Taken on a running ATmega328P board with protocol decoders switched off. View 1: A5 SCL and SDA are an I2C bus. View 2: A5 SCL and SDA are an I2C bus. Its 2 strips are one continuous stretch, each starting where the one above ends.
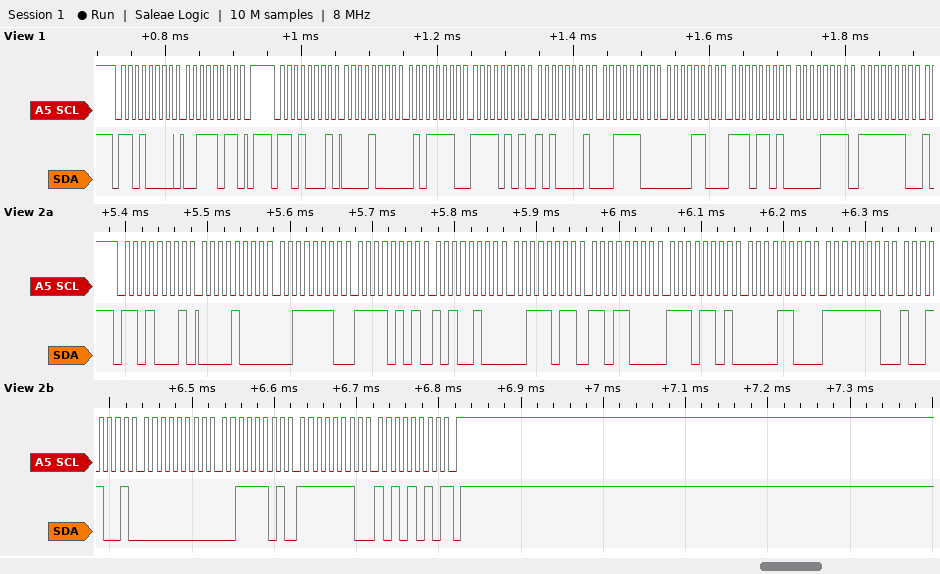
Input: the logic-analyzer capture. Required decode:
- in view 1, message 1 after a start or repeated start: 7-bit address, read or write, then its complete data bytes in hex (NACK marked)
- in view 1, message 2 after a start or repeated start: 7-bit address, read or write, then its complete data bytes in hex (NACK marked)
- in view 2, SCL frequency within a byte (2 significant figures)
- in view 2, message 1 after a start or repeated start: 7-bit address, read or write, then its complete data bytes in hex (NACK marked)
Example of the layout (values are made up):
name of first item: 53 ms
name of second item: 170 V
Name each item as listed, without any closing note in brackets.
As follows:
in view 1, message 1 after a start or repeated start: 7-bit address, read or write, then its complete data bytes in hex: 0x68 write: 3B
in view 1, message 2 after a start or repeated start: 7-bit address, read or write, then its complete data bytes in hex: 0x68 read: 08 5E F5 A1 3C 0C ED 0F FE
in view 2, SCL frequency within a byte: 100 kHz
in view 2, message 1 after a start or repeated start: 7-bit address, read or write, then its complete data bytes in hex: 0x68 read: 08 3E F5 A4 3B D8 ED 0C FE 99 00 3D FE AA NACK
